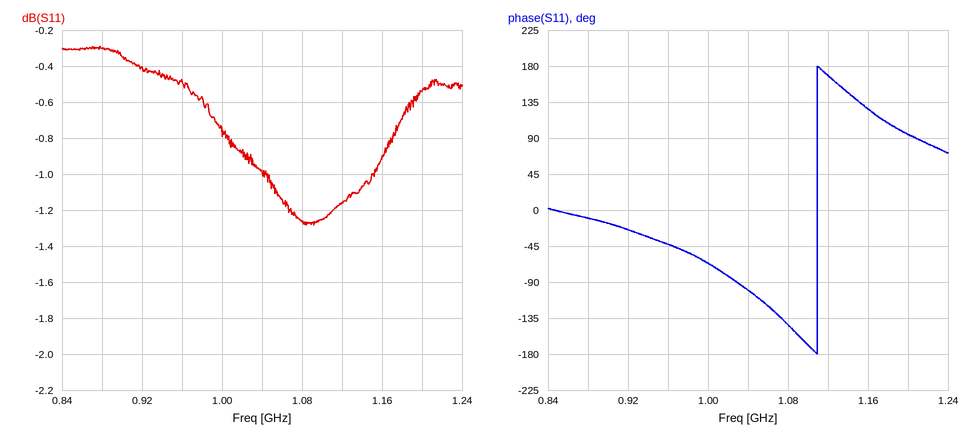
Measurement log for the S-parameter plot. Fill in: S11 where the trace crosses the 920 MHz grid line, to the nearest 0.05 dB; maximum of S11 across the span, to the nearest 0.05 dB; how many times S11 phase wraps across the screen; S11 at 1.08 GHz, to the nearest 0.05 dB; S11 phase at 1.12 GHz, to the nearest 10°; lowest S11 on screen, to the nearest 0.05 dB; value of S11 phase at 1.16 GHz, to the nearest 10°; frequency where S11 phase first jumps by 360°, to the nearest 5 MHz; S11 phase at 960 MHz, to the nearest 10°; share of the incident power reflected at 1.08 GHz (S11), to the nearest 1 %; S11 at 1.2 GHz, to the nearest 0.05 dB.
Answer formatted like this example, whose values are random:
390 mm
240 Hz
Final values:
-0.40 dB
-0.30 dB
1
-1.25 dB
170°
-1.30 dB
130°
1.110 GHz
-40°
75 %
-0.55 dB
